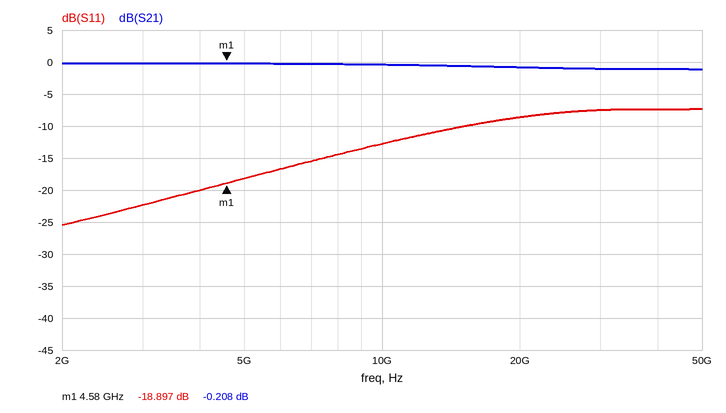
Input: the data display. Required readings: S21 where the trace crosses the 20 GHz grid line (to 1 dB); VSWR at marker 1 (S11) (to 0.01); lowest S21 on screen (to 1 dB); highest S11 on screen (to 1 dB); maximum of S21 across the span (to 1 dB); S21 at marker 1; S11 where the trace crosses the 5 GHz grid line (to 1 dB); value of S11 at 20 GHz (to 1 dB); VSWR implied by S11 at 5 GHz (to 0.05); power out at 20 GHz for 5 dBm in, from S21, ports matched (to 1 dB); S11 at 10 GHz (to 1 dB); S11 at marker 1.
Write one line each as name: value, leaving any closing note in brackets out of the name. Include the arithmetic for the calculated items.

S21 where the trace crosses the 20 GHz grid line: -1 dB
VSWR at marker 1 (S11): (1 + 0.1135)/(1 − 0.1135) ≈ 1.26
lowest S21 on screen: -1 dB
highest S11 on screen: -7 dB
maximum of S21 across the span: 0 dB
S21 at marker 1: -0.208 dB
S11 where the trace crosses the 5 GHz grid line: -18 dB
value of S11 at 20 GHz: -9 dB
VSWR implied by S11 at 5 GHz: |Γ| = 10^(-18/20) = 0.1259; VSWR = (1 + 0.1259)/(1 − 0.1259) ≈ 1.29, so 1.30 to the nearest 0.05
power out at 20 GHz for 5 dBm in, from S21, ports matched: 5 dBm + (-1 dB) = 4 dBm
S11 at 10 GHz: -13 dB
S11 at marker 1: -18.897 dB
